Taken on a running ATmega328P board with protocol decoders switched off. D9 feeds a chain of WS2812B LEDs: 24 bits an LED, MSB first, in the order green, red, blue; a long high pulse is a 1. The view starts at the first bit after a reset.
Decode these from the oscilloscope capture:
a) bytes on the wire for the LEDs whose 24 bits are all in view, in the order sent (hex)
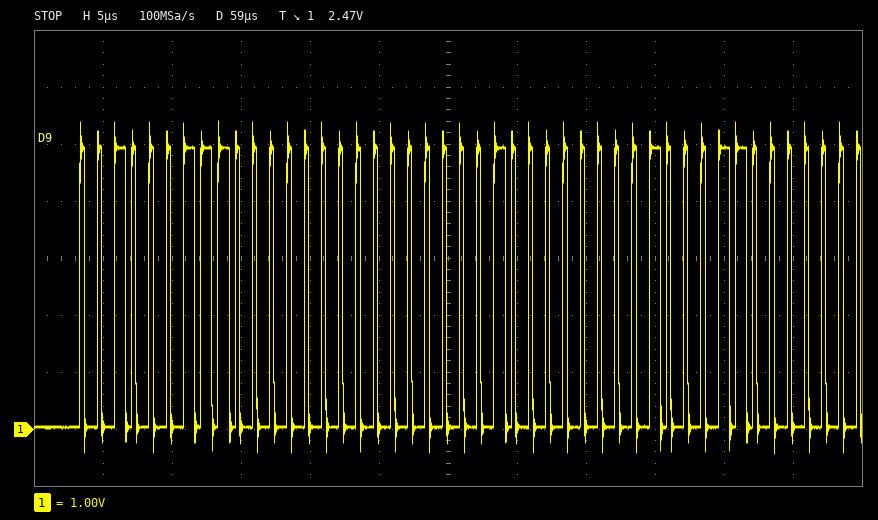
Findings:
23 80 00
